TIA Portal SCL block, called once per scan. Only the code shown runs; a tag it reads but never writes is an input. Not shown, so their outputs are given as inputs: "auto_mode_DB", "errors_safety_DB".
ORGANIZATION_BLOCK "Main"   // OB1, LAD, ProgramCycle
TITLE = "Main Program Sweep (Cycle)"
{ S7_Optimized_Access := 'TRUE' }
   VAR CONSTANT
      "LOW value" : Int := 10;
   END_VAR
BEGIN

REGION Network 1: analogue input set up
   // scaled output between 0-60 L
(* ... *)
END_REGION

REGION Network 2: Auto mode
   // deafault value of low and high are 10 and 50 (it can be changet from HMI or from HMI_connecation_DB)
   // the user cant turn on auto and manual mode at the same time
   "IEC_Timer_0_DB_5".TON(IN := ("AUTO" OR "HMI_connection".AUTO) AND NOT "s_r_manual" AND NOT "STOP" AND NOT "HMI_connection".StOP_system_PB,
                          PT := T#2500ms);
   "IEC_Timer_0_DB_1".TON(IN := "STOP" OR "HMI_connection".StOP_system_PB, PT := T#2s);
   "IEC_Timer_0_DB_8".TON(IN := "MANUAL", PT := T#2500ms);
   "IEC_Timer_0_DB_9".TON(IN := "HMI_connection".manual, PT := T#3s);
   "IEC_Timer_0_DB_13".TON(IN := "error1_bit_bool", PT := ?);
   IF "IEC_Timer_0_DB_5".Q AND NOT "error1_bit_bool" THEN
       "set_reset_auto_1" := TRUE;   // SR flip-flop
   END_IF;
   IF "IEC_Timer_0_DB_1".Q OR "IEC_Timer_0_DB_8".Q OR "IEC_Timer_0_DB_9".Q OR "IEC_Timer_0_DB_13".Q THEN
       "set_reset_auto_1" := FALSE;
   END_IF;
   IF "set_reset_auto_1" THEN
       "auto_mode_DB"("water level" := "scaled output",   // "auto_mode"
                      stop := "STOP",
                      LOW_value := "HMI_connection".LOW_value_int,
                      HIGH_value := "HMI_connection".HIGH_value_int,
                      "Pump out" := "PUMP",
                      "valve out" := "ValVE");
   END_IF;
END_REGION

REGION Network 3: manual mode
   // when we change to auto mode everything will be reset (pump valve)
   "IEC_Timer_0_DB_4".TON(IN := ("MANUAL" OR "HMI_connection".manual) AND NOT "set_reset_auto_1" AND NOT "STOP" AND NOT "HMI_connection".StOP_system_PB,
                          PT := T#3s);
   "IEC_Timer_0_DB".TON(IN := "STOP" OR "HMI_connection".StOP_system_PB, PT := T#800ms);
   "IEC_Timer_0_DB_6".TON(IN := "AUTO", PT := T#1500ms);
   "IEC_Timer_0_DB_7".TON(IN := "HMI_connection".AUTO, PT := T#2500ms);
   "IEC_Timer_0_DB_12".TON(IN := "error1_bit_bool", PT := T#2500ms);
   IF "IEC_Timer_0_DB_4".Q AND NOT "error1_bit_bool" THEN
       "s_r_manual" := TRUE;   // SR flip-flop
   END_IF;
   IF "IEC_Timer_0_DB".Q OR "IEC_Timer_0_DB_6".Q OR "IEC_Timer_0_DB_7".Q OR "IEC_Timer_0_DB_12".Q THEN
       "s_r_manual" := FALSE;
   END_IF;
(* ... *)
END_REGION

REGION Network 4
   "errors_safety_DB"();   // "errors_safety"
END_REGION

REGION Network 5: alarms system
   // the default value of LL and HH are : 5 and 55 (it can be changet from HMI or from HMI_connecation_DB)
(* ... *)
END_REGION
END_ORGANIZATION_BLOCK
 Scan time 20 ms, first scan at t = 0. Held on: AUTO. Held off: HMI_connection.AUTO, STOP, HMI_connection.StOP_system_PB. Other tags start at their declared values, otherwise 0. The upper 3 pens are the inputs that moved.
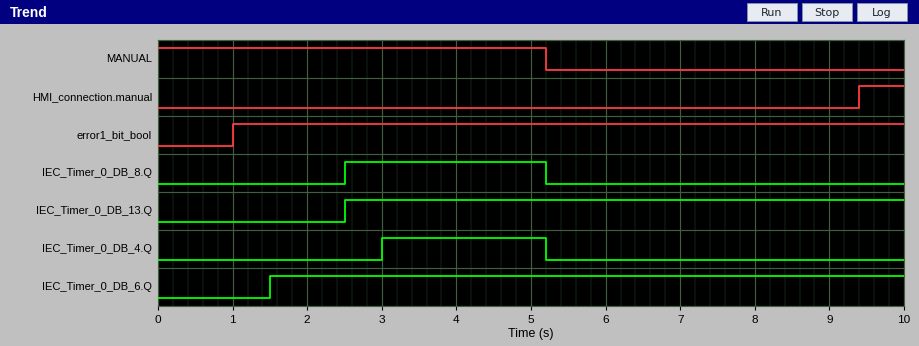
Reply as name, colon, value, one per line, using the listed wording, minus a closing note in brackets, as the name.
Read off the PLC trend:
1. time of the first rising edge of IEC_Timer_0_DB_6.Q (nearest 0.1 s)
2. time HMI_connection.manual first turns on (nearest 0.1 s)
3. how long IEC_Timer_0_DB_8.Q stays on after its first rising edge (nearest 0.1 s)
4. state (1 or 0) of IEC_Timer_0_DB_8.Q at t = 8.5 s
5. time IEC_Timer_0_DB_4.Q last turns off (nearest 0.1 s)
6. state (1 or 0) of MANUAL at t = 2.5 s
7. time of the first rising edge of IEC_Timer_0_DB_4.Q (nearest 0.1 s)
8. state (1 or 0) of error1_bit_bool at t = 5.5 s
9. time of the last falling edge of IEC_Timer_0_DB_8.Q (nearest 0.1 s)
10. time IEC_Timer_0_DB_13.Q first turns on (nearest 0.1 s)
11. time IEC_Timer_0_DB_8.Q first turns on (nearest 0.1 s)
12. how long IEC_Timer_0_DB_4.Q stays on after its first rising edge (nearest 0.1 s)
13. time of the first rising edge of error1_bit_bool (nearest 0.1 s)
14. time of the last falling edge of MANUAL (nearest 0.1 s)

time of the first rising edge of IEC_Timer_0_DB_6.Q: 1.5 s
time HMI_connection.manual first turns on: 9.4 s
how long IEC_Timer_0_DB_8.Q stays on after its first rising edge: 2.7 s
state (1 or 0) of IEC_Timer_0_DB_8.Q at t = 8.5 s: 0
time IEC_Timer_0_DB_4.Q last turns off: 5.2 s
state (1 or 0) of MANUAL at t = 2.5 s: 1
time of the first rising edge of IEC_Timer_0_DB_4.Q: 3.0 s
state (1 or 0) of error1_bit_bool at t = 5.5 s: 1
time of the last falling edge of IEC_Timer_0_DB_8.Q: 5.2 s
time IEC_Timer_0_DB_13.Q first turns on: 2.5 s
time IEC_Timer_0_DB_8.Q first turns on: 2.5 s
how long IEC_Timer_0_DB_4.Q stays on after its first rising edge: 2.2 s
time of the first rising edge of error1_bit_bool: 1.0 s
time of the last falling edge of MANUAL: 5.2 s
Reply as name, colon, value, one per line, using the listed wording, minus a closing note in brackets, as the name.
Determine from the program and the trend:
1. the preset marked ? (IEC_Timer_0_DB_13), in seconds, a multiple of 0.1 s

the preset marked ? (IEC_Timer_0_DB_13), in seconds, a multiple of 0.1 s: 1.5 s
